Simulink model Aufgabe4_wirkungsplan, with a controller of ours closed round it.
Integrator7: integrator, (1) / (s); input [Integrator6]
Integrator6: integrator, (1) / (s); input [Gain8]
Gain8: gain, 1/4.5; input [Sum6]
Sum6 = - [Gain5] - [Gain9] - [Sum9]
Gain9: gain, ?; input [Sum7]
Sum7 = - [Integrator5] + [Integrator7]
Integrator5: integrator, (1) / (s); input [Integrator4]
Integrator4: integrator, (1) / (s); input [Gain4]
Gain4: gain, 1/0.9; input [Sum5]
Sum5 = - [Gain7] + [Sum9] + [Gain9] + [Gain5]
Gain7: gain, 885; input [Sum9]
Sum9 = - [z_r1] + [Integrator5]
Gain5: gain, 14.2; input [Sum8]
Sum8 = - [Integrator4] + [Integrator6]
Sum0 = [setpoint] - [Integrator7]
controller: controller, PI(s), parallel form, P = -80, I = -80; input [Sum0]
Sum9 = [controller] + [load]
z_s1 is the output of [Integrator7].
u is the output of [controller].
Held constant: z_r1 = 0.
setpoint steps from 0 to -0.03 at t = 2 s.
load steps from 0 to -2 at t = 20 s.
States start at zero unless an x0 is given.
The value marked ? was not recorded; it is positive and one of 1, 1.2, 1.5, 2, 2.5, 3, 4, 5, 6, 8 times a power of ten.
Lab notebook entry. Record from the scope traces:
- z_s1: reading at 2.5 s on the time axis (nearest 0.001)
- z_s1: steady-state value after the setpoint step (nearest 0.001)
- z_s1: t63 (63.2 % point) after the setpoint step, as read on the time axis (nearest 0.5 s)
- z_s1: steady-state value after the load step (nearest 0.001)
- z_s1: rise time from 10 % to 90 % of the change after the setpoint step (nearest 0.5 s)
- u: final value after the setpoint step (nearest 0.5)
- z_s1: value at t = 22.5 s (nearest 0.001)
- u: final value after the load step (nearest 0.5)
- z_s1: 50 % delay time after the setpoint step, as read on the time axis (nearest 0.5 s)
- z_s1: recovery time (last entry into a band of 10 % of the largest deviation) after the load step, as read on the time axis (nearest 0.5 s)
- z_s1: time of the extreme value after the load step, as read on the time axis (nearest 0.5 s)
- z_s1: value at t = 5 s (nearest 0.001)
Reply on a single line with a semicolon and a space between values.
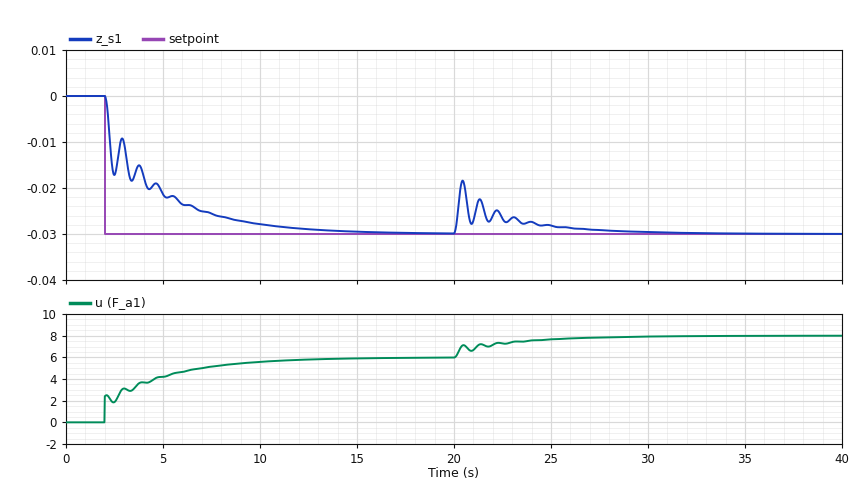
-0.017; -0.030; 4.0 s; -0.030; 6.5 s; 6.0; -0.027; 8.0; 2.5 s; 26.5 s; 20.5 s; -0.021
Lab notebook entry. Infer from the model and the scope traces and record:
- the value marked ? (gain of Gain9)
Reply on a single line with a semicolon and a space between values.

200
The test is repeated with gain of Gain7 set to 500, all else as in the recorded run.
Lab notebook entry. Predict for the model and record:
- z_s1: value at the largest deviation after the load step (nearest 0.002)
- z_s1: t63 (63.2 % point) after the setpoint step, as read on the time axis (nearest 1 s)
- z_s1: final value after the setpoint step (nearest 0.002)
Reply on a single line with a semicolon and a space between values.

-0.018; 3 s; -0.030
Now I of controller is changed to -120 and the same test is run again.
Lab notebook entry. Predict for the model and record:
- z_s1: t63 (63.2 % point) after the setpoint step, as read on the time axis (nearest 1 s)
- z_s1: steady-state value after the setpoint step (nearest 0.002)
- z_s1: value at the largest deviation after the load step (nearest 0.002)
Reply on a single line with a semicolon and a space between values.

3 s; -0.030; -0.018
